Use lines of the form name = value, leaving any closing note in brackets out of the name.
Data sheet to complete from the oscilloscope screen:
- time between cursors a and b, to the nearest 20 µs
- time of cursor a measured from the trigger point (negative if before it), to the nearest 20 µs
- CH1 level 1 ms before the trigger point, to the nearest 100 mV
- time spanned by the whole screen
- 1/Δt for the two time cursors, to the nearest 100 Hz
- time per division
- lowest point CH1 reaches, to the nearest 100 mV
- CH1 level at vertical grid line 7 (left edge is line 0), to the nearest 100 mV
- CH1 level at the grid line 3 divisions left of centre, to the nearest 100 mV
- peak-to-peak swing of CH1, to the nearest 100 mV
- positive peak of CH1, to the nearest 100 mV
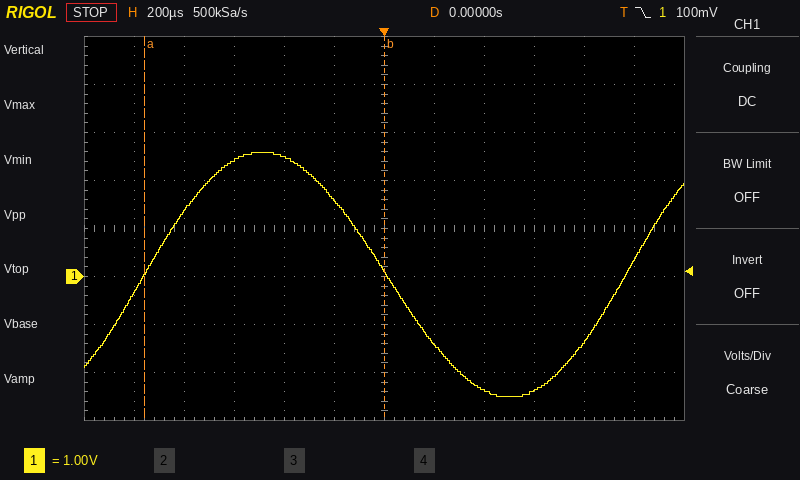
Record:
time between cursors a and b, to the nearest 20 µs = 960 µs
time of cursor a measured from the trigger point (negative if before it), to the nearest 20 µs = -960 µs
CH1 level 1 ms before the trigger point, to the nearest 100 mV = -300 mV
time spanned by the whole screen = 2.4 ms
1/Δt for the two time cursors, to the nearest 100 Hz = 1.0 kHz
time per division = 200 µs
lowest point CH1 reaches, to the nearest 100 mV = -2.5 V
CH1 level at vertical grid line 7 (left edge is line 0), to the nearest 100 mV = -1.4 V
CH1 level at the grid line 3 divisions left of centre, to the nearest 100 mV = 2.4 V
peak-to-peak swing of CH1, to the nearest 100 mV = 5.1 V
positive peak of CH1, to the nearest 100 mV = 2.6 V
